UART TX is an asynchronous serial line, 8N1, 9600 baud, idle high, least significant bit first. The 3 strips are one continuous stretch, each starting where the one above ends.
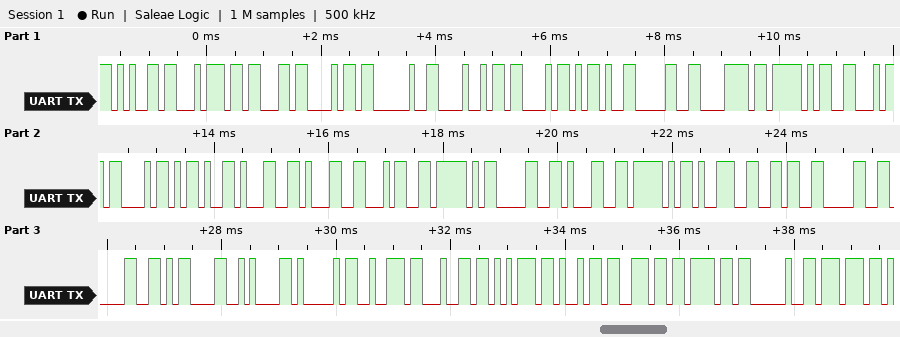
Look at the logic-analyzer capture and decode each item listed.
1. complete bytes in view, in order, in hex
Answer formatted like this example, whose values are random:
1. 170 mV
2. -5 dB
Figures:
1. 65 74 63 68 20 48 43 2D 30 78 5F 46 43 2D 31 31 34 5F 30 31 5F 39 36 30 30 0D 0A 41 72 64 75 69 6E 6F 20 77
